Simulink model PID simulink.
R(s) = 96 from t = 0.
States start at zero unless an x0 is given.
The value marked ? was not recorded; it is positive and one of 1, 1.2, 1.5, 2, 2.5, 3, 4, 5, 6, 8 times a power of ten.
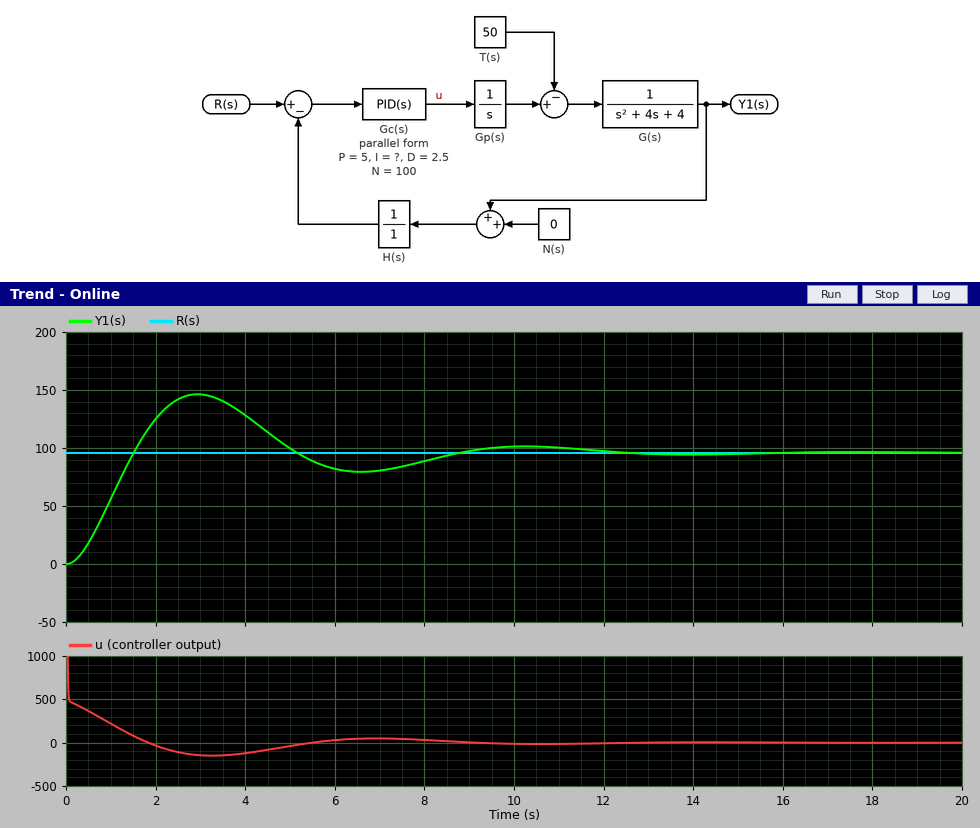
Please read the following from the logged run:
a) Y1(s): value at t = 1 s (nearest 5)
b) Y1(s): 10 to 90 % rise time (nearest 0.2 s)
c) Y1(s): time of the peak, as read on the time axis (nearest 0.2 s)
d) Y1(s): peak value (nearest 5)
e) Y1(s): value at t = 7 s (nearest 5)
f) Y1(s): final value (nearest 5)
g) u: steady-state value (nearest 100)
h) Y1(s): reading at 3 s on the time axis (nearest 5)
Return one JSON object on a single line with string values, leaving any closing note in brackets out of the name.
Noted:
{"Y1(s): value at t = 1 s": "55", "Y1(s): 10 to 90 % rise time": "1.0 s", "Y1(s): time of the peak, as read on the time axis": "3.0 s", "Y1(s): peak value": "145", "Y1(s): value at t = 7 s": "80", "Y1(s): final value": "95", "u: steady-state value": "0", "Y1(s): reading at 3 s on the time axis": "145"}
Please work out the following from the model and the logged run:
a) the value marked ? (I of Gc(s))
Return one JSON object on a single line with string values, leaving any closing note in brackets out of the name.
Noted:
{"the value marked ? (I of Gc(s))": "3"}
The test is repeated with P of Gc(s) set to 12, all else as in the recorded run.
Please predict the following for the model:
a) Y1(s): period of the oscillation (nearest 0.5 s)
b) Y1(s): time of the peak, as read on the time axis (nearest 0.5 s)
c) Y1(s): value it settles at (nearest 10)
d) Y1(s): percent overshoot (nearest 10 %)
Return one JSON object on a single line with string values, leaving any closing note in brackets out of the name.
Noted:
{"Y1(s): period of the oscillation": "3.5 s", "Y1(s): time of the peak, as read on the time axis": "2.0 s", "Y1(s): value it settles at": "100", "Y1(s): percent overshoot": "60 %"}
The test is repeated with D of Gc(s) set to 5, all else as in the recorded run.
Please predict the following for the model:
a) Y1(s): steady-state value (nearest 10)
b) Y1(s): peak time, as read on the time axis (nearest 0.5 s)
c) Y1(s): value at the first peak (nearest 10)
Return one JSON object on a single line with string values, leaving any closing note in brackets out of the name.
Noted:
{"Y1(s): steady-state value": "100", "Y1(s): peak time, as read on the time axis": "3.5 s", "Y1(s): value at the first peak": "120"}
